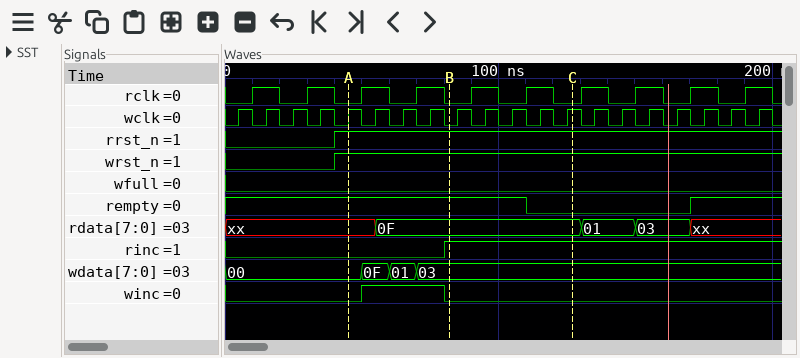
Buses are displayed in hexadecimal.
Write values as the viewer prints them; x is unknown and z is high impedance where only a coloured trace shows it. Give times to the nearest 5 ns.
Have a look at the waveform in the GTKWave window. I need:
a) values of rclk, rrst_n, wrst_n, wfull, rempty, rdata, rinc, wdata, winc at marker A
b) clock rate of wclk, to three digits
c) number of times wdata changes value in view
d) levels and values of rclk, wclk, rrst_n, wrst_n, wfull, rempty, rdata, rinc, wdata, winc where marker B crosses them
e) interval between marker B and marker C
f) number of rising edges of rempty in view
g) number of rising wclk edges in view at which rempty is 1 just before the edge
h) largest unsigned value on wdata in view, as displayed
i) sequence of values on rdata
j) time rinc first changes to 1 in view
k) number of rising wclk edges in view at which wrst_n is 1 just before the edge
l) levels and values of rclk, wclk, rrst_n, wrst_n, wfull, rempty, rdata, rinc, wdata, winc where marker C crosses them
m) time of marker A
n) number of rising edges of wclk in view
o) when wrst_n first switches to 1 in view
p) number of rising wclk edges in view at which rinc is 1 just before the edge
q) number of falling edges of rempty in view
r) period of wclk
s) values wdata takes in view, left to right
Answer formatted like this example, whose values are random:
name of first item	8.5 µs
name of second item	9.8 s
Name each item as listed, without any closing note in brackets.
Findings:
values of rclk, rrst_n, wrst_n, wfull, rempty, rdata, rinc, wdata, winc at marker A	rclk=0, rrst_n=1, wrst_n=1, wfull=0, rempty=1, rdata=xx, rinc=0, wdata=00, winc=0
clock rate of wclk, to three digits	100 MHz
number of times wdata changes value in view	3
levels and values of rclk, wclk, rrst_n, wrst_n, wfull, rempty, rdata, rinc, wdata, winc where marker B crosses them	rclk=0, wclk=0, rrst_n=1, wrst_n=1, wfull=0, rempty=1, rdata=0F, rinc=1, wdata=03, winc=0
interval between marker B and marker C	45 ns
number of rising edges of rempty in view	1
number of rising wclk edges in view at which rempty is 1 just before the edge	14
largest unsigned value on wdata in view, as displayed	0F
sequence of values on rdata	xx, 0F, 01, 03, xx
time rinc first changes to 1 in view	80 ns
number of rising wclk edges in view at which wrst_n is 1 just before the edge	16
levels and values of rclk, wclk, rrst_n, wrst_n, wfull, rempty, rdata, rinc, wdata, winc where marker C crosses them	rclk=0, wclk=1, rrst_n=1, wrst_n=1, wfull=0, rempty=0, rdata=0F, rinc=1, wdata=03, winc=0
time of marker A	45 ns
number of rising edges of wclk in view	20
when wrst_n first switches to 1 in view	40 ns
number of rising wclk edges in view at which rinc is 1 just before the edge	12
number of falling edges of rempty in view	1
period of wclk	10 ns
values wdata takes in view, left to right	00, 0F, 01, 03
